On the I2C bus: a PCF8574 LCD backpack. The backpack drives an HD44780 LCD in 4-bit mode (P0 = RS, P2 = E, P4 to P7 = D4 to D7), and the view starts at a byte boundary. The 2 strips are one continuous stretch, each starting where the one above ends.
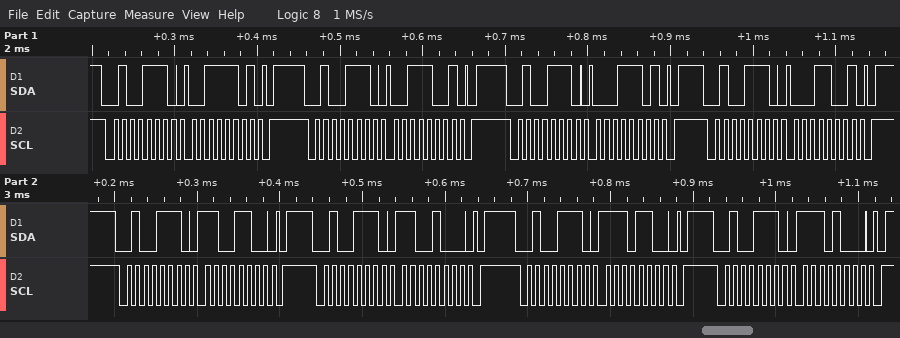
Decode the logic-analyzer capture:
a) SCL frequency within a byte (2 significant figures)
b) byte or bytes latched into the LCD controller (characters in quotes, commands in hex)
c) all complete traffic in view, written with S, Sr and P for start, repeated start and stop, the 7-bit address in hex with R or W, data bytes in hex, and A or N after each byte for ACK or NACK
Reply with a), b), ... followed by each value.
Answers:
a) 100 kHz
b) '1' 0xCE
c) S 27W A 3D A P S 27W A 39 A P S 27W A 1D A P S 27W A 19 A P S 27W A CC A P S 27W A C8 A P S 27W A EC A P S 27W A E8 A P
